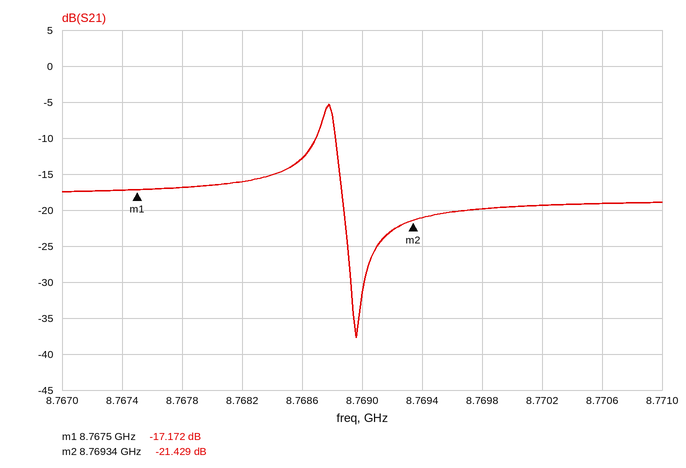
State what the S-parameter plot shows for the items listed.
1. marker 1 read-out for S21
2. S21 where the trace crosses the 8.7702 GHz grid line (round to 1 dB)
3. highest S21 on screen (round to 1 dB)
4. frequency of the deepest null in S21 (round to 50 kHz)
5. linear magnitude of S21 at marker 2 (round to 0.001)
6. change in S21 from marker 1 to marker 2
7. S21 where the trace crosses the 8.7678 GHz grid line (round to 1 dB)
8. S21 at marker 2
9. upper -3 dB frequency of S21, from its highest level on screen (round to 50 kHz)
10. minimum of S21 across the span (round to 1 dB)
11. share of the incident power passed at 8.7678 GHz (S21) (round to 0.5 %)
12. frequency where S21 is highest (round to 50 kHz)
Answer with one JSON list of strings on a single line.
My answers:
["-17.172 dB", "-19 dB", "-5 dB", "8.76895 GHz", "0.085", "-4.257 dB", "-17 dB", "-21.429 dB", "8.76880 GHz", "-38 dB", "2.0 %", "8.76880 GHz"]
